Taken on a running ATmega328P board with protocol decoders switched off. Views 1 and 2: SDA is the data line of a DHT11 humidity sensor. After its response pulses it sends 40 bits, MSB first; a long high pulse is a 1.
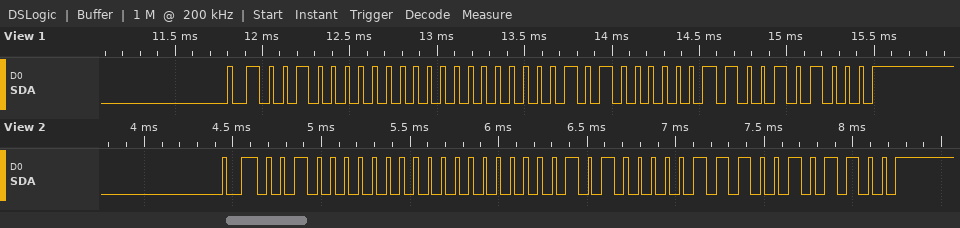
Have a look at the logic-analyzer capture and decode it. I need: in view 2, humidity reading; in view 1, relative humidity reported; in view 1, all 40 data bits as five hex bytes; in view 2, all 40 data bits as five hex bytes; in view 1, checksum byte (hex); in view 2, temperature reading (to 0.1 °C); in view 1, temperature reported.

32 %
32 %
20 00 05 03 28
20 00 05 07 2C
0x28
5.7 °C
5.3 °C
